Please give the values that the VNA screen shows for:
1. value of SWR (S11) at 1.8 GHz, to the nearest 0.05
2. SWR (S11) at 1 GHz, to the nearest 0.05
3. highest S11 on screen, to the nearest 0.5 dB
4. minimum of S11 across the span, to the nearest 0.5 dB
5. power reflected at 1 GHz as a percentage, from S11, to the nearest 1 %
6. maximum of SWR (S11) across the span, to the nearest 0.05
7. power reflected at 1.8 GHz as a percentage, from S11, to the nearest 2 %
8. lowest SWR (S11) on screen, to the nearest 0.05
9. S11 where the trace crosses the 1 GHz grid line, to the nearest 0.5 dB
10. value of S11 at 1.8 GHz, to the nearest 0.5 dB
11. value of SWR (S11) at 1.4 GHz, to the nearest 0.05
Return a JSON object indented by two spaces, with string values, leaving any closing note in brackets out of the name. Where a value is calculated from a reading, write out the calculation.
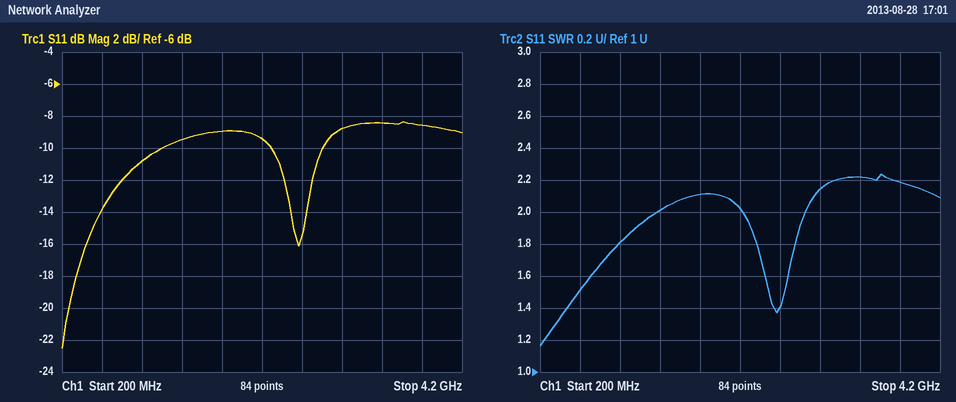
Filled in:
{
  "value of SWR (S11) at 1.8 GHz, to the nearest 0.05": "2.10",
  "SWR (S11) at 1 GHz, to the nearest 0.05": "1.80",
  "highest S11 on screen, to the nearest 0.5 dB": "-8.5 dB",
  "minimum of S11 across the span, to the nearest 0.5 dB": "-22.5 dB",
  "power reflected at 1 GHz as a percentage, from S11, to the nearest 1 %": "10^(-11/10) ≈ 8 %",
  "maximum of SWR (S11) across the span, to the nearest 0.05": "2.25",
  "power reflected at 1.8 GHz as a percentage, from S11, to the nearest 2 %": "10^(-9/10) ≈ 12.6 %, so 12 % to the nearest 2 %",
  "lowest SWR (S11) on screen, to the nearest 0.05": "1.15",
  "S11 where the trace crosses the 1 GHz grid line, to the nearest 0.5 dB": "-11.0 dB",
  "value of S11 at 1.8 GHz, to the nearest 0.5 dB": "-9.0 dB",
  "value of SWR (S11) at 1.4 GHz, to the nearest 0.05": "2.00"
}
